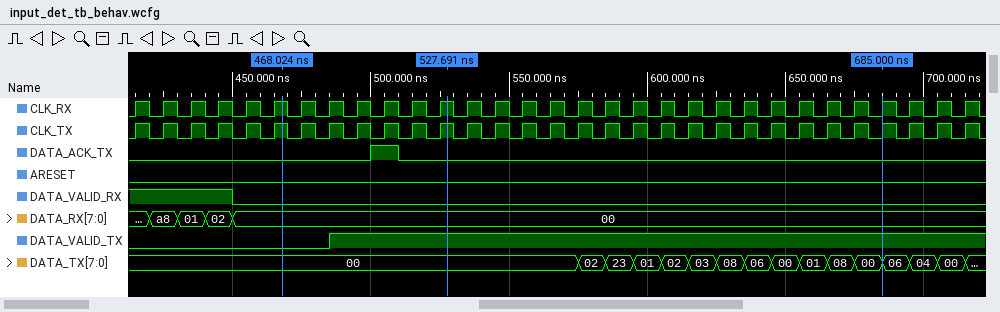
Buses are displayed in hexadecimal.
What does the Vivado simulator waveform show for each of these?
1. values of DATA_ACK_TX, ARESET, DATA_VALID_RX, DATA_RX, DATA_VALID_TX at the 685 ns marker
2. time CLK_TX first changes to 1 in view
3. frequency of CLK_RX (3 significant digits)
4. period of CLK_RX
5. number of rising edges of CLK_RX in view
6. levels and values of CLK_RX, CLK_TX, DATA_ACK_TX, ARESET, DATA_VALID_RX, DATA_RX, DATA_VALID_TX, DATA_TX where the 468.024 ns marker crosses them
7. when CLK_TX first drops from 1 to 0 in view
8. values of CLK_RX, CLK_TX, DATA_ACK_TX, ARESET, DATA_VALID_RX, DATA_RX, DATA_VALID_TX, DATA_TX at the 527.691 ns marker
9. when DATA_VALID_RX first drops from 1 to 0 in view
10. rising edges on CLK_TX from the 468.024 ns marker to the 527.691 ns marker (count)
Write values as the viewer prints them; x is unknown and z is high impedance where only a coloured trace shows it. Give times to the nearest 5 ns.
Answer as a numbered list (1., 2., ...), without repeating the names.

1. DATA_ACK_TX=0, ARESET=0, DATA_VALID_RX=0, DATA_RX=00, DATA_VALID_TX=1
2. 415 ns
3. 100 MHz
4. 10 ns
5. 31
6. CLK_RX=1, CLK_TX=1, DATA_ACK_TX=0, ARESET=0, DATA_VALID_RX=0, DATA_RX=00, DATA_VALID_TX=0, DATA_TX=00
7. 420 ns
8. CLK_RX=1, CLK_TX=1, DATA_ACK_TX=0, ARESET=0, DATA_VALID_RX=0, DATA_RX=00, DATA_VALID_TX=1, DATA_TX=00
9. 450 ns
10. 6
